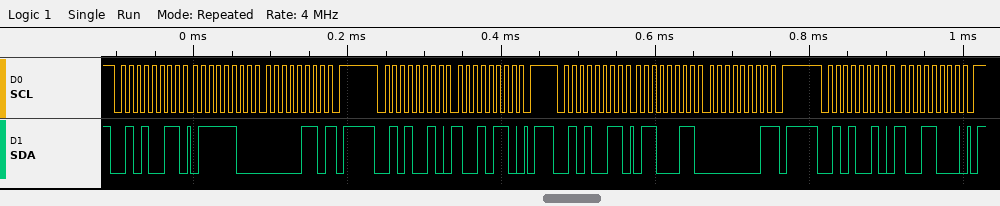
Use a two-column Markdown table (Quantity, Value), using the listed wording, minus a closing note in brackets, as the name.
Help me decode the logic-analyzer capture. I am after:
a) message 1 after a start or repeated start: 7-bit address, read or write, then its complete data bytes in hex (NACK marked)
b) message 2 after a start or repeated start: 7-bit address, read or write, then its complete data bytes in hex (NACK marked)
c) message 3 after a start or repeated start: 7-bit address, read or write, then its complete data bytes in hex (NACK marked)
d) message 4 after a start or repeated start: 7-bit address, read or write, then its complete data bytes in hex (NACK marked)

| Quantity | Value |
|---|---|
| message 1 after a start or repeated start: 7-bit address, read or write, then its complete data bytes in hex | 0x29 read: 7C 06 NACK |
| message 2 after a start or repeated start: 7-bit address, read or write, then its complete data bytes in hex | 0x29 write: 96 |
| message 3 after a start or repeated start: 7-bit address, read or write, then its complete data bytes in hex | 0x29 read: 63 01 NACK |
| message 4 after a start or repeated start: 7-bit address, read or write, then its complete data bytes in hex | 0x29 write: 98 |
